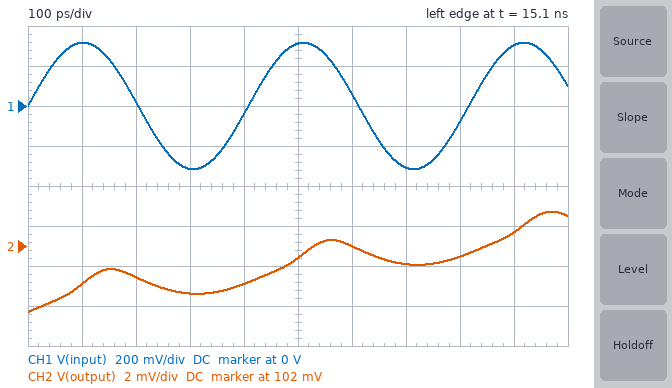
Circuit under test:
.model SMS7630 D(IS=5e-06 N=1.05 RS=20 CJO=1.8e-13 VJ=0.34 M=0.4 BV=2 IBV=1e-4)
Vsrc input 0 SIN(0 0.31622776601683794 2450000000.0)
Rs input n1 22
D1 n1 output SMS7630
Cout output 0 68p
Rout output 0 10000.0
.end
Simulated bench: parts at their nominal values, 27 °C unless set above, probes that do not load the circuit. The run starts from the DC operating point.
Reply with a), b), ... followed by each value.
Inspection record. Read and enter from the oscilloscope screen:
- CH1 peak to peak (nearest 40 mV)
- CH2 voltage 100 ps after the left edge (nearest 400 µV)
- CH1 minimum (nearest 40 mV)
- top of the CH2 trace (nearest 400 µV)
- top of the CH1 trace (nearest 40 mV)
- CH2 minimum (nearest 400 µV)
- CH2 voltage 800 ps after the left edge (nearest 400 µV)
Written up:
a) 640 mV
b) 100.0 mV
c) -320 mV
d) 103.6 mV
e) 320 mV
f) 98.8 mV
g) 101.6 mV
